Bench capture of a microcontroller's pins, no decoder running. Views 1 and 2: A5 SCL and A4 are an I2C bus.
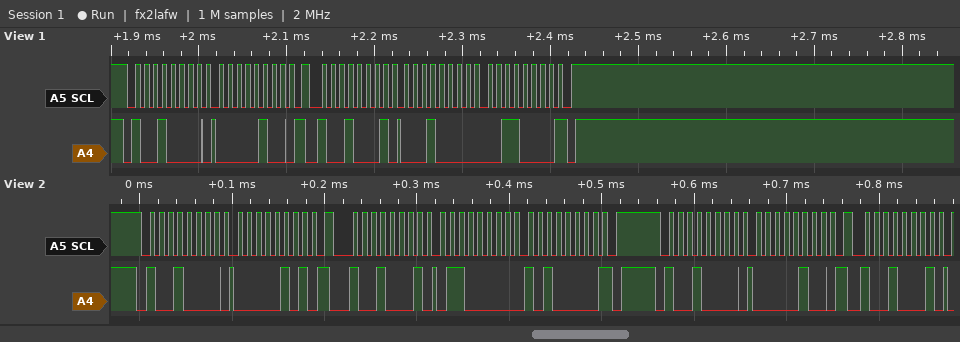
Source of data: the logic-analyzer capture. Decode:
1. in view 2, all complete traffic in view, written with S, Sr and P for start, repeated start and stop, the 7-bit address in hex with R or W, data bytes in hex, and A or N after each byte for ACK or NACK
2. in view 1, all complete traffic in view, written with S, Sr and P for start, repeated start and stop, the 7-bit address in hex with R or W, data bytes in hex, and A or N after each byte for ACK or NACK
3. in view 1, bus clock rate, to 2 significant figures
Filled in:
S 48W A 05 A Sr 48R A 60 A A0 N P S 48W A 04 A Sr 48R A
S 48W A 04 A Sr 48R A 10 A 30 N P
100 kHz
